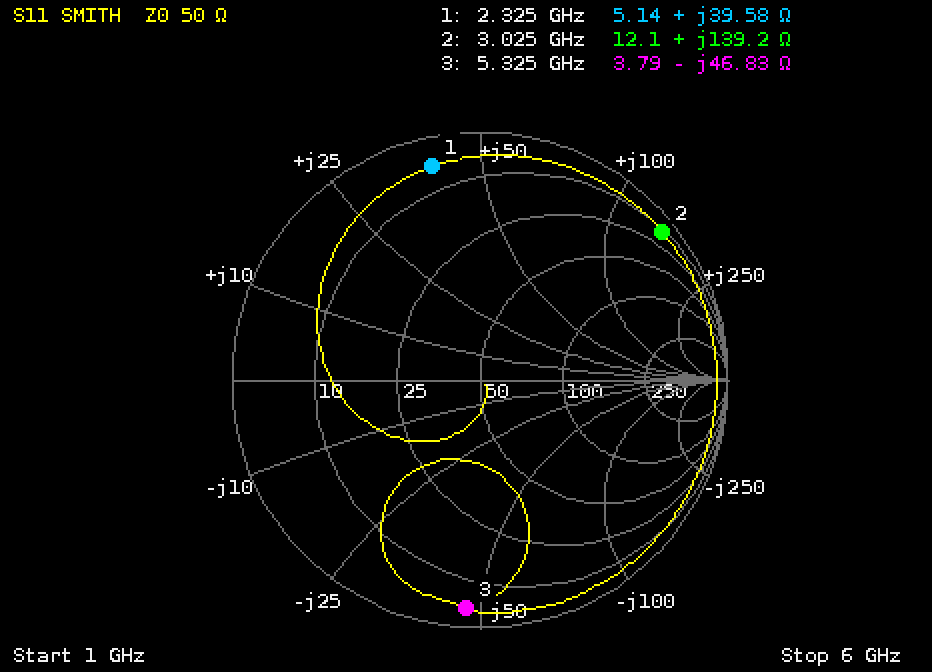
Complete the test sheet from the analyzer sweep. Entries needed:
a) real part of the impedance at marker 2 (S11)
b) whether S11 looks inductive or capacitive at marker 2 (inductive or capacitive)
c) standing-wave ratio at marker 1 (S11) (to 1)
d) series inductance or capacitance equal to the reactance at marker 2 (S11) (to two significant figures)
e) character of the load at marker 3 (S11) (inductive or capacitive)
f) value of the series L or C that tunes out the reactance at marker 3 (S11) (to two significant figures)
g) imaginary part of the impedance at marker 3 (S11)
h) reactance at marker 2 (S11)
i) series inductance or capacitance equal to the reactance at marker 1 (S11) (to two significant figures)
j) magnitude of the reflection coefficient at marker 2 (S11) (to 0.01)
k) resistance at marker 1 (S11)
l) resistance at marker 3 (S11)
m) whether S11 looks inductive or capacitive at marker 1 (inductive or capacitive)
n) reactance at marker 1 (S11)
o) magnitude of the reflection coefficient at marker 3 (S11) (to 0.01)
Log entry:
12.1 Ω
inductive
16
7.3 nH
capacitive
1.4 nH
-46.83 Ω
+139.2 Ω
2.7 nH
0.95
5.14 Ω
3.79 Ω
inductive
+39.58 Ω
0.92
